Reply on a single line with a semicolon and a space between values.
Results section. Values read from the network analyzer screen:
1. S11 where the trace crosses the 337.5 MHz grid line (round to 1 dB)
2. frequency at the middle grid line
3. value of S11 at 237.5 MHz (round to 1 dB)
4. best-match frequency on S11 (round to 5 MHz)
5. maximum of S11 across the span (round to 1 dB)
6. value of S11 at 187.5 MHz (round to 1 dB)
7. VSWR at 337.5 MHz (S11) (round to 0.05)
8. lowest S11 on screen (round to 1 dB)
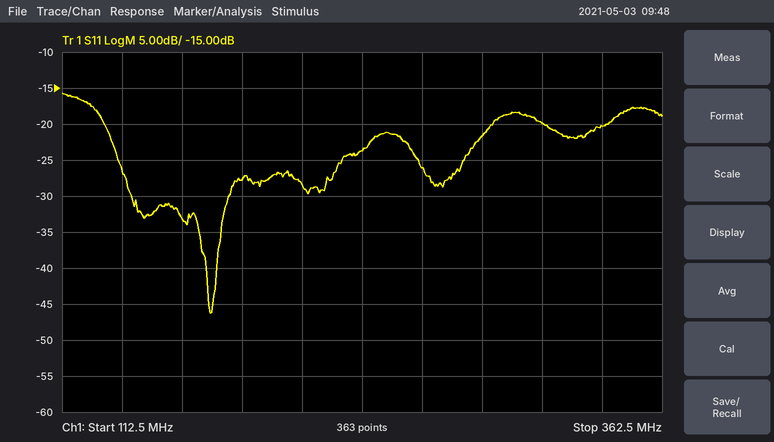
-20 dB; 237.5 MHz; -24 dB; 175 MHz; -16 dB; -28 dB; 1.20; -46 dB
